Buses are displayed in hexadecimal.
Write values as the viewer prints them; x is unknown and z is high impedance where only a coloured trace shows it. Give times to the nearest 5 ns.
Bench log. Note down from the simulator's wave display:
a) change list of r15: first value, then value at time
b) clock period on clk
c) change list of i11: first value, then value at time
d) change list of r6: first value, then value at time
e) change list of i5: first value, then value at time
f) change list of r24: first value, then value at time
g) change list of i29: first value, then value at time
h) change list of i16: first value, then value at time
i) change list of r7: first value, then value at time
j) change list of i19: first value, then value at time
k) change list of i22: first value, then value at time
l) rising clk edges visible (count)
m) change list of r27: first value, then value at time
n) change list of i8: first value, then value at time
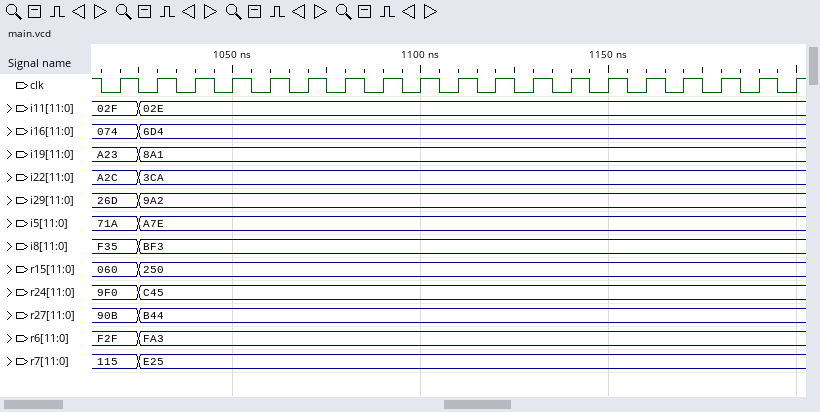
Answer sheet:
060, 250 at 1025 ns
10 ns
02F, 02E at 1025 ns
F2F, FA3 at 1025 ns
71A, A7E at 1025 ns
9F0, C45 at 1025 ns
26D, 9A2 at 1025 ns
074, 6D4 at 1025 ns
115, E25 at 1025 ns
A23, 8A1 at 1025 ns
A2C, 3CA at 1025 ns
19
90B, B44 at 1025 ns
F35, BF3 at 1025 ns
